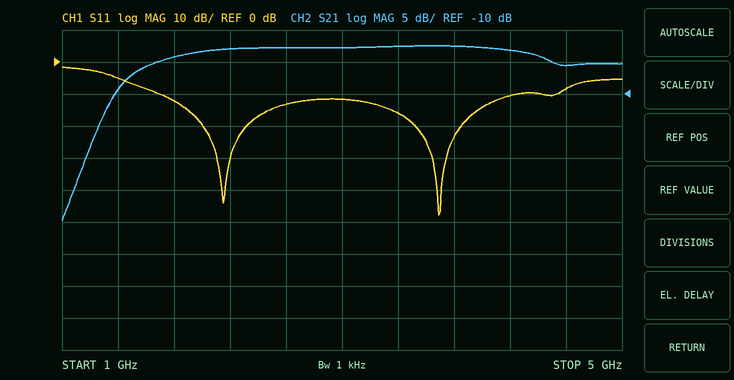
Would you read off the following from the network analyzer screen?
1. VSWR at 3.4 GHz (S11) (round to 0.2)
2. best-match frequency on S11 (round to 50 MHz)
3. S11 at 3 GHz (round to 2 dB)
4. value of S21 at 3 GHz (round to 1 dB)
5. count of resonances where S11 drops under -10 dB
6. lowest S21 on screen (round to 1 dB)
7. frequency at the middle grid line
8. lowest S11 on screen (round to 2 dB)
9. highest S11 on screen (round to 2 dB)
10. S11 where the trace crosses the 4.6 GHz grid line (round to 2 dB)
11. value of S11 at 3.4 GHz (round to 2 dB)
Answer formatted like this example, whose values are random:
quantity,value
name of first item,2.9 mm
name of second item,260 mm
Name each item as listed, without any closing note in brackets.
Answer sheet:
quantity,value
VSWR at 3.4 GHz (S11),1.4
best-match frequency on S11,3.70 GHz
S11 at 3 GHz,-12 dB
value of S21 at 3 GHz,-3 dB
count of resonances where S11 drops under -10 dB,2
lowest S21 on screen,-30 dB
frequency at the middle grid line,3 GHz
lowest S11 on screen,-48 dB
highest S11 on screen,-2 dB
S11 where the trace crosses the 4.6 GHz grid line,-8 dB
value of S11 at 3.4 GHz,-16 dB
